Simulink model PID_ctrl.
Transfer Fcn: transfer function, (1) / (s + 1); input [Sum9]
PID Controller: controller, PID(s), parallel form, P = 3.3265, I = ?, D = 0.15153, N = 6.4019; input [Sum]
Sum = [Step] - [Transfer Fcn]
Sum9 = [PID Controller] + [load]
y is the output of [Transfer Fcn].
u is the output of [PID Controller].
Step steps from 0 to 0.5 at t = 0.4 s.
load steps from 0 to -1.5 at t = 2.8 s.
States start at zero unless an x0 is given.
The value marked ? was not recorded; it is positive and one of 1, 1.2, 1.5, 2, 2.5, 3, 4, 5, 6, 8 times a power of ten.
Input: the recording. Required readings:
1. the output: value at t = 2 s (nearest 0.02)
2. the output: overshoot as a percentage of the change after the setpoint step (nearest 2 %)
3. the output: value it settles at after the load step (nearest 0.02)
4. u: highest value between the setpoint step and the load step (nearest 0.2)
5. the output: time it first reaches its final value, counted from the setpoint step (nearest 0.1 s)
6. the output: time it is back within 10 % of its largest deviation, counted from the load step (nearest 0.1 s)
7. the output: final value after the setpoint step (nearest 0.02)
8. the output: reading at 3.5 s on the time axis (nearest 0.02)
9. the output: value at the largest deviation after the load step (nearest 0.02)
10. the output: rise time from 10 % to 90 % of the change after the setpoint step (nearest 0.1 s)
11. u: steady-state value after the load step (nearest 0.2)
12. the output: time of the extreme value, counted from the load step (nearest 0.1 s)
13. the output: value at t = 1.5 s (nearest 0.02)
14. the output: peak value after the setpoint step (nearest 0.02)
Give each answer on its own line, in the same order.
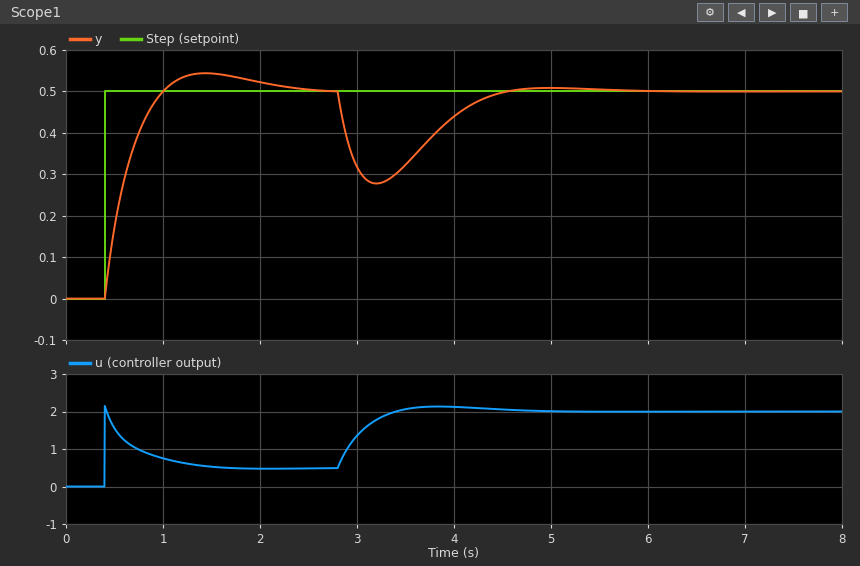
0.52
8 %
0.50
2.2
0.6 s
1.5 s
0.50
0.32
0.28
0.4 s
2.0
0.4 s
0.54
0.54
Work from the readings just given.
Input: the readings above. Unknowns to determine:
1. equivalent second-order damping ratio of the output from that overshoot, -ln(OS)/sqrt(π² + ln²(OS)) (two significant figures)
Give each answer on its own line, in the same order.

0.63
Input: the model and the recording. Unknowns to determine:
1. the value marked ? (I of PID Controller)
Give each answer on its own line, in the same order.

8
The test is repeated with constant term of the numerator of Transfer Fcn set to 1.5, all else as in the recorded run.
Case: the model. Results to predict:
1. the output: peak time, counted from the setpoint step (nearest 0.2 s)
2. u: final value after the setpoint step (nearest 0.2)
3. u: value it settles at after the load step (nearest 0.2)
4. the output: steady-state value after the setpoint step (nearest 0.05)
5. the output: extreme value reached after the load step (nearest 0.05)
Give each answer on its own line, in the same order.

0.8 s
0.4
1.8
0.50
0.25
